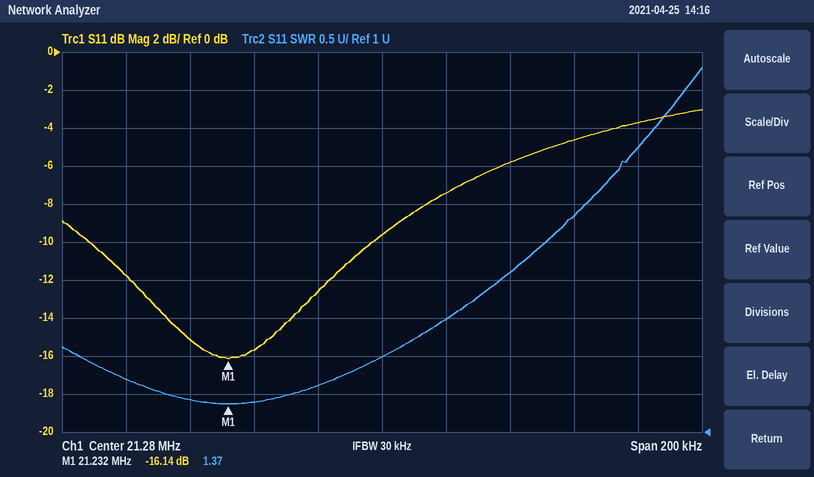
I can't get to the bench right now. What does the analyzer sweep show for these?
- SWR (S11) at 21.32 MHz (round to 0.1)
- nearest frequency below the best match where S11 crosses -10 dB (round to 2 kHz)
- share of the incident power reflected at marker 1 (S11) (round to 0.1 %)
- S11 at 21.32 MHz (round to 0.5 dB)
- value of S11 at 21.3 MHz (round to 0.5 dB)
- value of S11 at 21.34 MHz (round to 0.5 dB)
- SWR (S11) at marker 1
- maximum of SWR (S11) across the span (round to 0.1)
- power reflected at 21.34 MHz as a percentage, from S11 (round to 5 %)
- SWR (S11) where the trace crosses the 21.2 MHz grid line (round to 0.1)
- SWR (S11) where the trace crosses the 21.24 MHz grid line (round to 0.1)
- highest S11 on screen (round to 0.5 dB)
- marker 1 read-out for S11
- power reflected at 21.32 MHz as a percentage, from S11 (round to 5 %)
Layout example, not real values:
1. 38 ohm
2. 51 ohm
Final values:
1. 3.1
2. 21.188 MHz
3. 2.4 %
4. -6.0 dB
5. -7.5 dB
6. -4.5 dB
7. 1.37
8. 5.8
9. 35 %
10. 1.7
11. 1.4
12. -3.0 dB
13. -16.14 dB
14. 25 %
